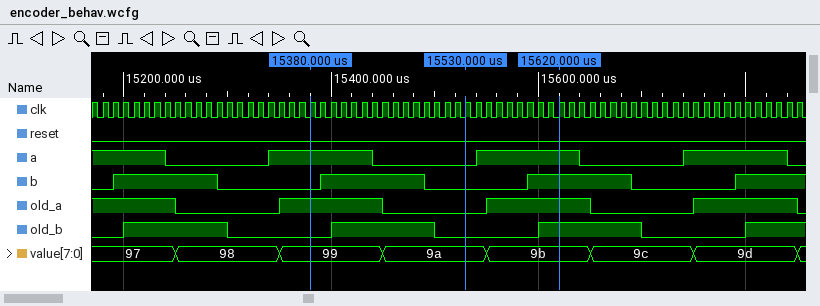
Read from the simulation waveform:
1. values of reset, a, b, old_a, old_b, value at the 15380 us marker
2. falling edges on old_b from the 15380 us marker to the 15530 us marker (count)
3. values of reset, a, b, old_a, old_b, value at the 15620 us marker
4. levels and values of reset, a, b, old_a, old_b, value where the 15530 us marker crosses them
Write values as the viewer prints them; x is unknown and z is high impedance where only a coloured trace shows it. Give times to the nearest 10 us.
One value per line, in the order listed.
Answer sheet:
reset=0, a=1, b=0, old_a=1, old_b=0, value=99
1
reset=0, a=1, b=1, old_a=1, old_b=1, value=9b
reset=0, a=0, b=0, old_a=0, old_b=0, value=9a
